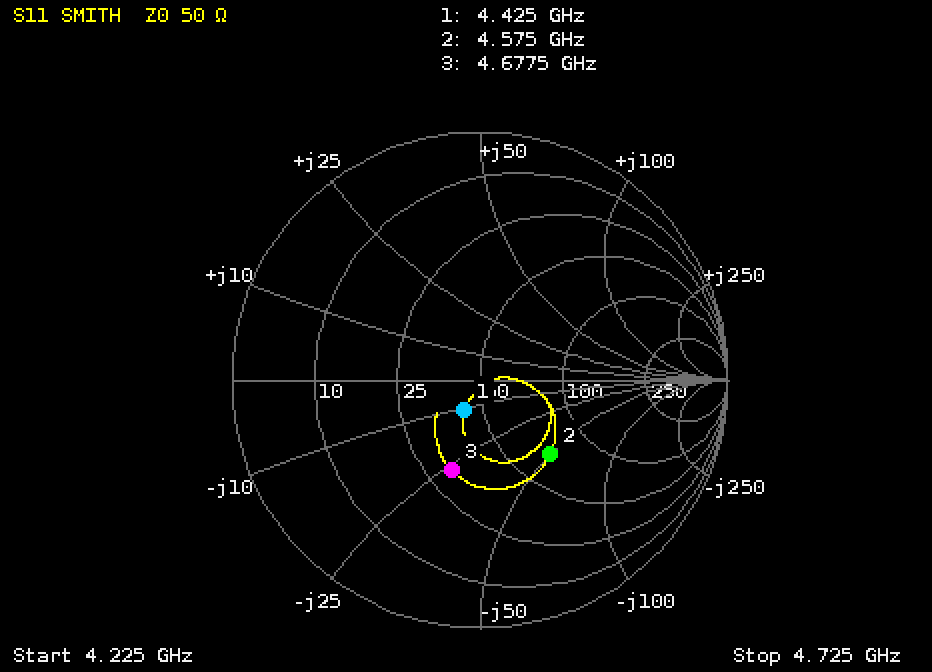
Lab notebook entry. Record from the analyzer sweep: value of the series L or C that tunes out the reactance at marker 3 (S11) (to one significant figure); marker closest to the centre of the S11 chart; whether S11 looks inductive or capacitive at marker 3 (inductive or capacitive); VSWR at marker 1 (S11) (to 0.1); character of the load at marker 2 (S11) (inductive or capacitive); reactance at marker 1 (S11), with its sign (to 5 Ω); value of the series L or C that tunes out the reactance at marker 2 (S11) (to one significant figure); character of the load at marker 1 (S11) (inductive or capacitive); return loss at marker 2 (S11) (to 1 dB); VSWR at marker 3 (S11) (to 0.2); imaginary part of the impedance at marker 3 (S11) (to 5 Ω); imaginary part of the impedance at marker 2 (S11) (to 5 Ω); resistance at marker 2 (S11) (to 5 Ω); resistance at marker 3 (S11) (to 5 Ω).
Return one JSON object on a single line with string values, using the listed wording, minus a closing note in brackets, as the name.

{"value of the series L or C that tunes out the reactance at marker 3 (S11)": "900 pH", "marker closest to the centre of the S11 chart": "marker 1", "whether S11 looks inductive or capacitive at marker 3": "capacitive", "VSWR at marker 1 (S11)": "1.3", "character of the load at marker 2 (S11)": "capacitive", "reactance at marker 1 (S11), with its sign": "-10 Ω", "value of the series L or C that tunes out the reactance at marker 2 (S11)": "2 nH", "character of the load at marker 1 (S11)": "capacitive", "return loss at marker 2 (S11)": "8 dB", "VSWR at marker 3 (S11)": "2.2", "imaginary part of the impedance at marker 3 (S11)": "-25 Ω", "imaginary part of the impedance at marker 2 (S11)": "-50 Ω", "resistance at marker 2 (S11)": "70 Ω", "resistance at marker 3 (S11)": "30 Ω"}
